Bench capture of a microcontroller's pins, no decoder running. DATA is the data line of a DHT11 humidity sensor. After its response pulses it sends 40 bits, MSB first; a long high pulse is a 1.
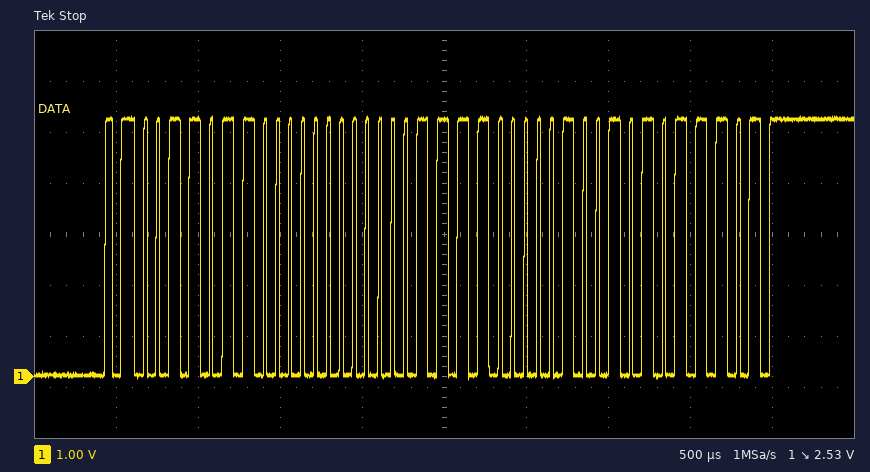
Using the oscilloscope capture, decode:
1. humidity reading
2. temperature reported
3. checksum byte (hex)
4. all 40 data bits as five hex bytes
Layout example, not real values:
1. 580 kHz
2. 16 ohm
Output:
1. 54 %
2. 30.9 °C
3. 0x5D
4. 36 00 1E 09 5D
